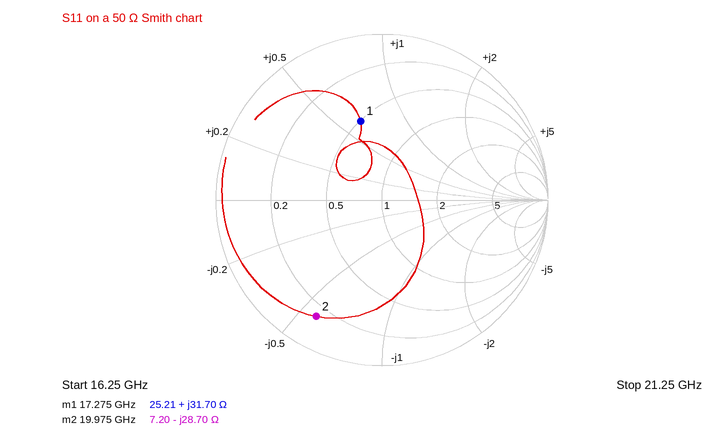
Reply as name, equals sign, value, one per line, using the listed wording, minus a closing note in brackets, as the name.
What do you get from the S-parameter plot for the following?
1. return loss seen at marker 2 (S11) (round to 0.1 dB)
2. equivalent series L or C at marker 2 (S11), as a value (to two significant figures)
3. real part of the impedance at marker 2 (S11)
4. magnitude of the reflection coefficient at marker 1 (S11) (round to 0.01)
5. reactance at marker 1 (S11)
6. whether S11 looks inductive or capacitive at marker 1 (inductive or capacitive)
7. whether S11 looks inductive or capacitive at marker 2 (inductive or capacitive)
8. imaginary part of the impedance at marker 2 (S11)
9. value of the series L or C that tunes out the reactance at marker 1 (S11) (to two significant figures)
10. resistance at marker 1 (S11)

return loss seen at marker 2 (S11) = 1.9 dB
equivalent series L or C at marker 2 (S11), as a value = 280 fF
real part of the impedance at marker 2 = 7.20 Ω
magnitude of the reflection coefficient at marker 1 (S11) = 0.49
reactance at marker 1 = +31.70 Ω
whether S11 looks inductive or capacitive at marker 1 = inductive
whether S11 looks inductive or capacitive at marker 2 = capacitive
imaginary part of the impedance at marker 2 = -28.70 Ω
value of the series L or C that tunes out the reactance at marker 1 (S11) = 290 fF
resistance at marker 1 = 25.21 Ω
